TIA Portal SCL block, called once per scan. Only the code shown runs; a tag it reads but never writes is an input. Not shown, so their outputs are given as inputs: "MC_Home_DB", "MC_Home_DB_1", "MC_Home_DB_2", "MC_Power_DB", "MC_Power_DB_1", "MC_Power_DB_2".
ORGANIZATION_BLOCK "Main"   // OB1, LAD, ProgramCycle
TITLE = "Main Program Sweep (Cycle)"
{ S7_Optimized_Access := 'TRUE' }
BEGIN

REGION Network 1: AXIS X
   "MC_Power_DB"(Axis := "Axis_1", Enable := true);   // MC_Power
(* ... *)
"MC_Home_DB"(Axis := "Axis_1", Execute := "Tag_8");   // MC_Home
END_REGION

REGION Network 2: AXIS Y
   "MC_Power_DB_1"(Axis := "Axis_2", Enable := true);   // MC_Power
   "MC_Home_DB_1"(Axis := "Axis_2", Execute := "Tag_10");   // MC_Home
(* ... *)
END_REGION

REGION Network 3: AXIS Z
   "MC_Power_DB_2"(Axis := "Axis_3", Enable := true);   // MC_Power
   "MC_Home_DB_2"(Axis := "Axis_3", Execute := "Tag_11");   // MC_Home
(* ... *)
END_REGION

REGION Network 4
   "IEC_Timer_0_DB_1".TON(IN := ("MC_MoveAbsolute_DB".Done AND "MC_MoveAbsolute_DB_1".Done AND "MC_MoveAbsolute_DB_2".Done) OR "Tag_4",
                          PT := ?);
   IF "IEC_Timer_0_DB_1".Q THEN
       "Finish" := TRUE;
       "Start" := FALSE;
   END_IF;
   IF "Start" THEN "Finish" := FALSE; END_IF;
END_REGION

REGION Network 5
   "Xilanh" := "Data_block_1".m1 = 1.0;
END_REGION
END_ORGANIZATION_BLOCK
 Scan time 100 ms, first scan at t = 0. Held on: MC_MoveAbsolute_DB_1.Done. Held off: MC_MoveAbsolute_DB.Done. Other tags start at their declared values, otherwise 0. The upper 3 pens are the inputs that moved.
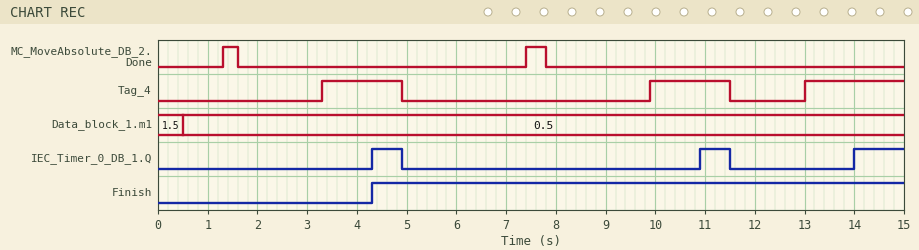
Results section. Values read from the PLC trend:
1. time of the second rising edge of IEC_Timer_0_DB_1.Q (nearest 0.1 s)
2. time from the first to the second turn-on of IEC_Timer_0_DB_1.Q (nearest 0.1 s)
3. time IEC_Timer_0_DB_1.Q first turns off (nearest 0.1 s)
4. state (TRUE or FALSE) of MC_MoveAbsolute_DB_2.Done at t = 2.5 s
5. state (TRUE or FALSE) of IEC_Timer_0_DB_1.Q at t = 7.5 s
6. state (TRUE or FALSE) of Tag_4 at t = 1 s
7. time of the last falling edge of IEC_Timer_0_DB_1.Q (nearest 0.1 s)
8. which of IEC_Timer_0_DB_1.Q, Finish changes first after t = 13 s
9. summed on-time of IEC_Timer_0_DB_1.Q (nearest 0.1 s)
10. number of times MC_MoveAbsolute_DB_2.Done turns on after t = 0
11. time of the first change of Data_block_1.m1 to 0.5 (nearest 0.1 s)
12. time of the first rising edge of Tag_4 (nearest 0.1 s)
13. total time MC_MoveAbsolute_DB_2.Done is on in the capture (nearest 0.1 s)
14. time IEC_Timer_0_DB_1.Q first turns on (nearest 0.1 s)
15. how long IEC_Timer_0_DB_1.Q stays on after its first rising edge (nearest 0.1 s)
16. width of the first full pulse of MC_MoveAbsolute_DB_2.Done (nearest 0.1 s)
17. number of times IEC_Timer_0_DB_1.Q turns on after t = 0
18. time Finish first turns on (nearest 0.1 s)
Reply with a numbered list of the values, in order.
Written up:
1. 10.9 s
2. 6.6 s
3. 4.9 s
4. FALSE
5. FALSE
6. FALSE
7. 11.5 s
8. IEC_Timer_0_DB_1.Q
9. 2.2 s
10. 2
11. 0.5 s
12. 3.3 s
13. 0.7 s
14. 4.3 s
15. 0.6 s
16. 0.3 s
17. 3
18. 4.3 s
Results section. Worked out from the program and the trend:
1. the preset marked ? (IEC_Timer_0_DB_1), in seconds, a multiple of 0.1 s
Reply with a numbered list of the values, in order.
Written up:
1. 1.0 s
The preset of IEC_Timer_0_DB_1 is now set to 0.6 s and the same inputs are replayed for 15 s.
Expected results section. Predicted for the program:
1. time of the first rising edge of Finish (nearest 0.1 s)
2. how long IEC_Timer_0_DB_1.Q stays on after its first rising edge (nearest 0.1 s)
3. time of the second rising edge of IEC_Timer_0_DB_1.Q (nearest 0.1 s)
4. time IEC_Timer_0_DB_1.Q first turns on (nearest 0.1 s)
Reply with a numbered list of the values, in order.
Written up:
1. 3.9 s
2. 1.0 s
3. 10.5 s
4. 3.9 s
